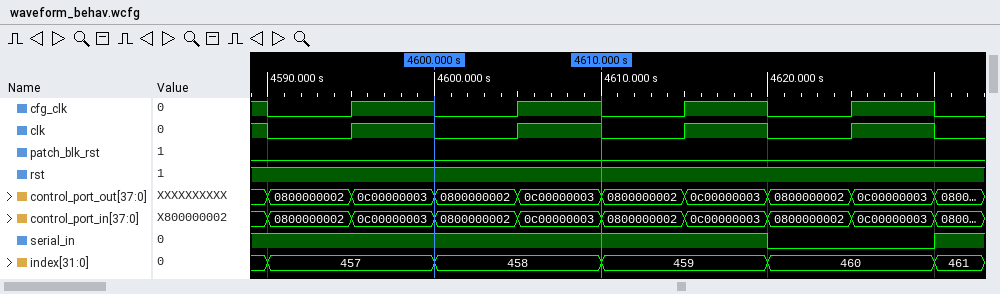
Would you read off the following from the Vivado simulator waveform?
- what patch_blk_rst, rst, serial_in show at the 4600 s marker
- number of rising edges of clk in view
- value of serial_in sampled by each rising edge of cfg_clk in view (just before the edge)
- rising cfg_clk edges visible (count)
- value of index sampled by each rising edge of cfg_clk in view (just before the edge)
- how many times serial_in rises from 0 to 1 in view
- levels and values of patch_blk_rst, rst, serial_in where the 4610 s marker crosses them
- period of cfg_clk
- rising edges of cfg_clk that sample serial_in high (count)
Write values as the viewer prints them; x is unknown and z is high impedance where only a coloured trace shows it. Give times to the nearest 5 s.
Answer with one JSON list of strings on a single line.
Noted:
["patch_blk_rst=0, rst=1, serial_in=1", "4", "1 1 1 0", "4", "457, 458, 459, 460", "1", "patch_blk_rst=0, rst=1, serial_in=1", "10 s", "3"]
